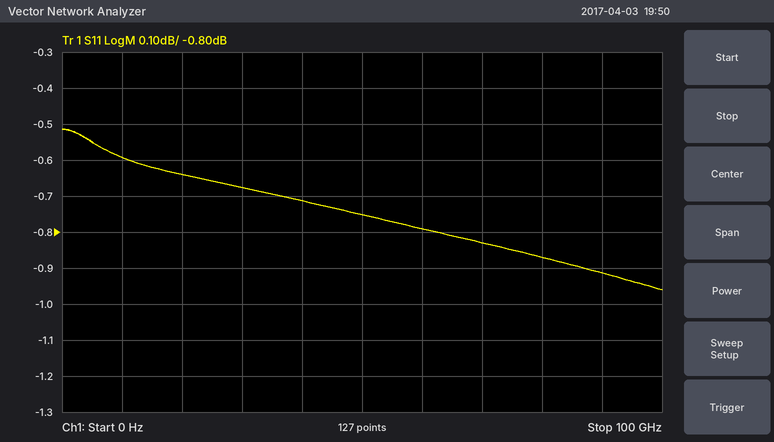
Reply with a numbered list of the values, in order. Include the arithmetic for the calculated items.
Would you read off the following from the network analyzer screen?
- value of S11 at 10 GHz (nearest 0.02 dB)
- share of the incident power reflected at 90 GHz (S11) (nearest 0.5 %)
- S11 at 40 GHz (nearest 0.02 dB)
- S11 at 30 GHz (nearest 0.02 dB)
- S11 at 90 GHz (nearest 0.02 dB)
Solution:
1. -0.60 dB
2. 10^(-0.92/10) ≈ 80.9 %, so 81.0 % to the nearest 0.5 %
3. -0.72 dB
4. -0.68 dB
5. -0.92 dB
